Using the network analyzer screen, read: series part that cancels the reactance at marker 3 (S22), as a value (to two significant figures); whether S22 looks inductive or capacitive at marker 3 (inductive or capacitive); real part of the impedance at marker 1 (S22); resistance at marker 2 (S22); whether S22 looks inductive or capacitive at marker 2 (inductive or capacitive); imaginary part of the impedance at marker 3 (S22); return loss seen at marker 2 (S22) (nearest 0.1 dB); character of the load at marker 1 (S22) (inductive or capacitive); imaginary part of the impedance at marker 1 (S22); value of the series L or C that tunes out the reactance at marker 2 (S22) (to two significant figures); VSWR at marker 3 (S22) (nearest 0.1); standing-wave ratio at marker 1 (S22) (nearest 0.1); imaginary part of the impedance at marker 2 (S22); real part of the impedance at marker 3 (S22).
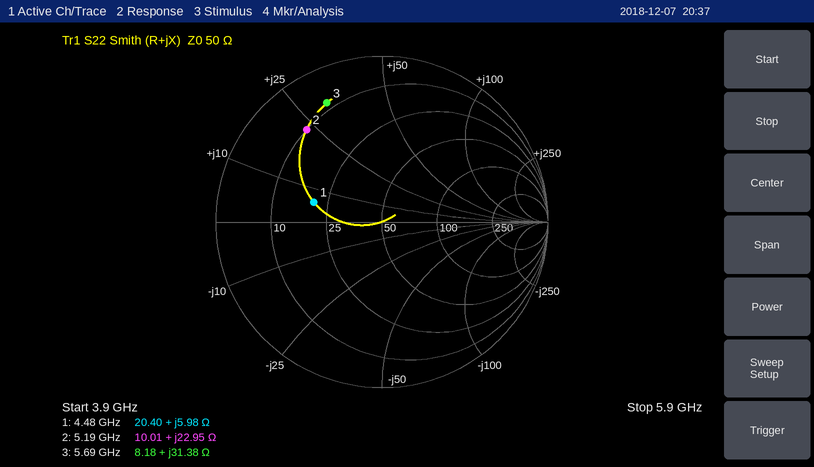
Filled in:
890 fF
inductive
20.40 Ω
10.01 Ω
inductive
+31.38 Ω
2.9 dB
inductive
+5.98 Ω
1.3 pF
8.6
2.5
+22.95 Ω
8.18 Ω
